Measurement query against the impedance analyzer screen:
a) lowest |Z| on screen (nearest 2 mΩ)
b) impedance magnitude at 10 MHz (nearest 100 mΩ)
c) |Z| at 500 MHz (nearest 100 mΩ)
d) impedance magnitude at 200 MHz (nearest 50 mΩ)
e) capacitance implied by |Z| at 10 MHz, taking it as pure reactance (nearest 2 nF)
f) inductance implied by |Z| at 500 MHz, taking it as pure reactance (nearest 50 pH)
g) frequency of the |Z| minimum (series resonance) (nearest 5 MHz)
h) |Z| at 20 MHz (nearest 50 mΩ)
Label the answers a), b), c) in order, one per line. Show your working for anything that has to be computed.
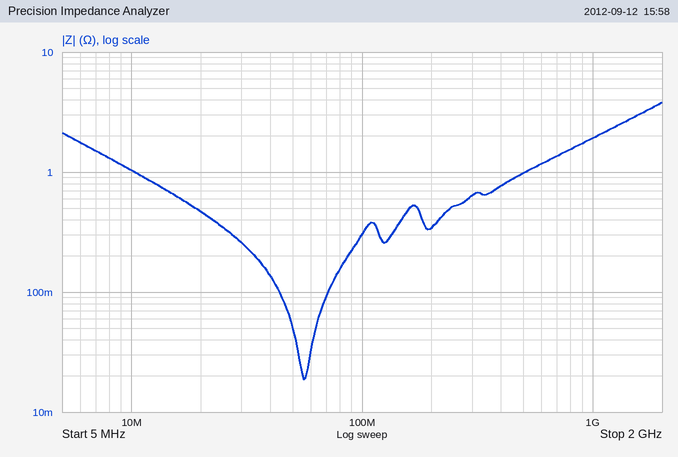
a) 18 mΩ
b) 1.0 Ω
c) 1.0 Ω
d) 350 mΩ
e) C = 1/(2π × 10 MHz × 1.0 Ω) ≈ 16 nF
f) L = 1.0 Ω/(2π × 500 MHz) ≈ 318 pH, so 300 pH to the nearest 50 pH
g) 55 MHz
h) 450 mΩ
